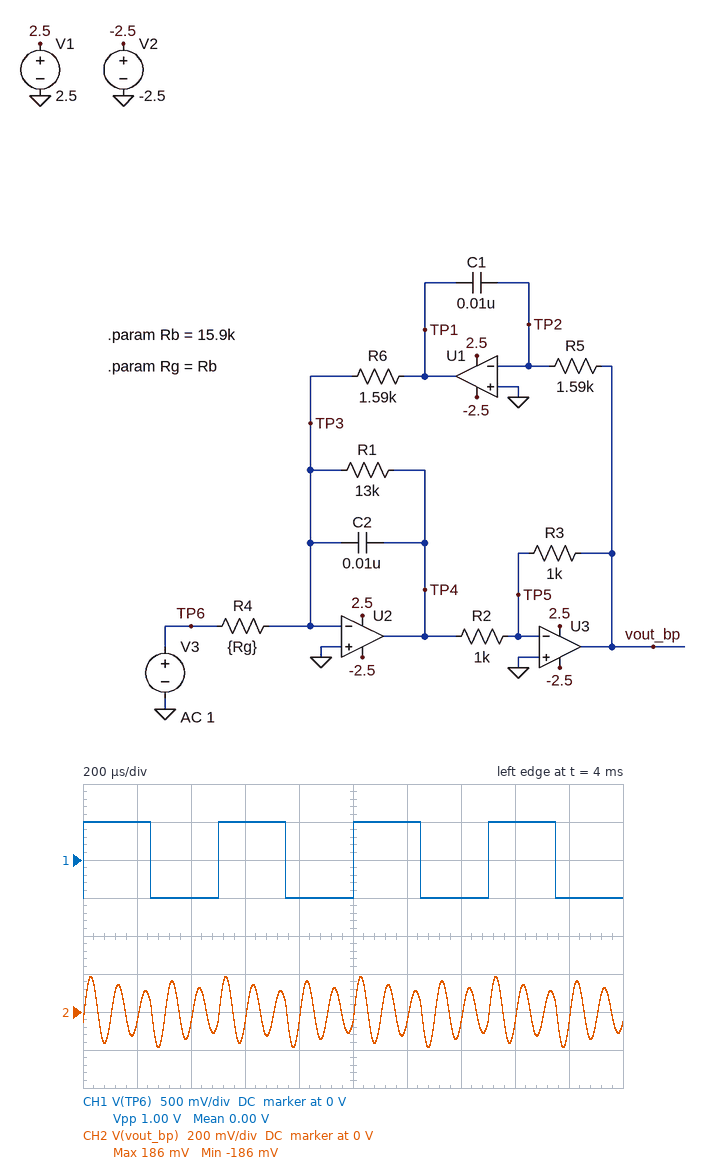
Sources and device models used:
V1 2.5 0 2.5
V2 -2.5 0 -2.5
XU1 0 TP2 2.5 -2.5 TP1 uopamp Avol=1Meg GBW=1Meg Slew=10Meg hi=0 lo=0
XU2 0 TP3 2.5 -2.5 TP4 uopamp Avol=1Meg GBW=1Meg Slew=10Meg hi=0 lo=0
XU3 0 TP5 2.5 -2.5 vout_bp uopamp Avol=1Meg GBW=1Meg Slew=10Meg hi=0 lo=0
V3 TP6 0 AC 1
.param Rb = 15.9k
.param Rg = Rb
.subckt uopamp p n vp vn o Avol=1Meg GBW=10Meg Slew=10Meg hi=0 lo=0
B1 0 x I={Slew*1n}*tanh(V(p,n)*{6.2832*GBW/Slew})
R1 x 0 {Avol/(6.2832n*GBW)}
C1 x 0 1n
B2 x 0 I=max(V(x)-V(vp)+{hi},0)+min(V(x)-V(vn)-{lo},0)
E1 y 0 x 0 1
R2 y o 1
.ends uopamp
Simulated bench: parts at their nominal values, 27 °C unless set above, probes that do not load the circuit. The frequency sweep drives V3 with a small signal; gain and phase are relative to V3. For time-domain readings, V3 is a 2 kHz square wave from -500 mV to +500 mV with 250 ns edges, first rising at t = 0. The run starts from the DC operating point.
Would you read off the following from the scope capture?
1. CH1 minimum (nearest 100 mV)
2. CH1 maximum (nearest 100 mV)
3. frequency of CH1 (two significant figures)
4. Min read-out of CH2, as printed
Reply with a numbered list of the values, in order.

1. -500 mV
2. 500 mV
3. 2.0 kHz
4. -186 mV
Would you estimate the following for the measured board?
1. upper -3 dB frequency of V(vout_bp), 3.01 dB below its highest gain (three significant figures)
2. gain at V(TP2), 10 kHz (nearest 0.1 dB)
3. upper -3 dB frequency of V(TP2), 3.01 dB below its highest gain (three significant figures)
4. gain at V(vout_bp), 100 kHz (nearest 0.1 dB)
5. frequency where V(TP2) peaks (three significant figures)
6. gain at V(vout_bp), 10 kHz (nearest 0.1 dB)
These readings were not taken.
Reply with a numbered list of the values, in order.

1. 10.3 kHz
2. -38.7 dB
3. 10.3 kHz
4. -40.2 dB
5. 9.90 kHz
6. 1.4 dB
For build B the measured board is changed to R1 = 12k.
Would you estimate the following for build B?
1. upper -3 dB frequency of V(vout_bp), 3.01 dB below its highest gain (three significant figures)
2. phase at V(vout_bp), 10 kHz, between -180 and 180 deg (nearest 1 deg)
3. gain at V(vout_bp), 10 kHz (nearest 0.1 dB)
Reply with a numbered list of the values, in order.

1. 10.4 kHz
2. -14 deg
3. 0.4 dB
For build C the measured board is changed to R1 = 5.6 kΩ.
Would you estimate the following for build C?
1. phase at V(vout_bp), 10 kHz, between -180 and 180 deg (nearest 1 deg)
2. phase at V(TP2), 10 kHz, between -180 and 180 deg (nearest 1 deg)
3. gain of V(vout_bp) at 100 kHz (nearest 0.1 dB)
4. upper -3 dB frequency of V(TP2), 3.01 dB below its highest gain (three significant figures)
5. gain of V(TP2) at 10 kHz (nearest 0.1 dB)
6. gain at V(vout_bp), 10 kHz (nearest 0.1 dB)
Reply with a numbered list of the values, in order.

1. -6 deg
2. -7 deg
3. -40.2 dB
4. 11.2 kHz
5. -47.9 dB
6. -7.8 dB
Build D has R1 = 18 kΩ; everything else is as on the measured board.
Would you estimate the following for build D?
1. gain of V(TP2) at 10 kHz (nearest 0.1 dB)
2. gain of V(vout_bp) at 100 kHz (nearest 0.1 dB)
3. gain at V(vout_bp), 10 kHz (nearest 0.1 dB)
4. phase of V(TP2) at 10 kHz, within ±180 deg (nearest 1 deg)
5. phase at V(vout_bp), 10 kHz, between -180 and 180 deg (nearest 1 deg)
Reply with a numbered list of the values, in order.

1. -34.5 dB
2. -40.2 dB
3. 5.5 dB
4. -25 deg
5. -24 deg
